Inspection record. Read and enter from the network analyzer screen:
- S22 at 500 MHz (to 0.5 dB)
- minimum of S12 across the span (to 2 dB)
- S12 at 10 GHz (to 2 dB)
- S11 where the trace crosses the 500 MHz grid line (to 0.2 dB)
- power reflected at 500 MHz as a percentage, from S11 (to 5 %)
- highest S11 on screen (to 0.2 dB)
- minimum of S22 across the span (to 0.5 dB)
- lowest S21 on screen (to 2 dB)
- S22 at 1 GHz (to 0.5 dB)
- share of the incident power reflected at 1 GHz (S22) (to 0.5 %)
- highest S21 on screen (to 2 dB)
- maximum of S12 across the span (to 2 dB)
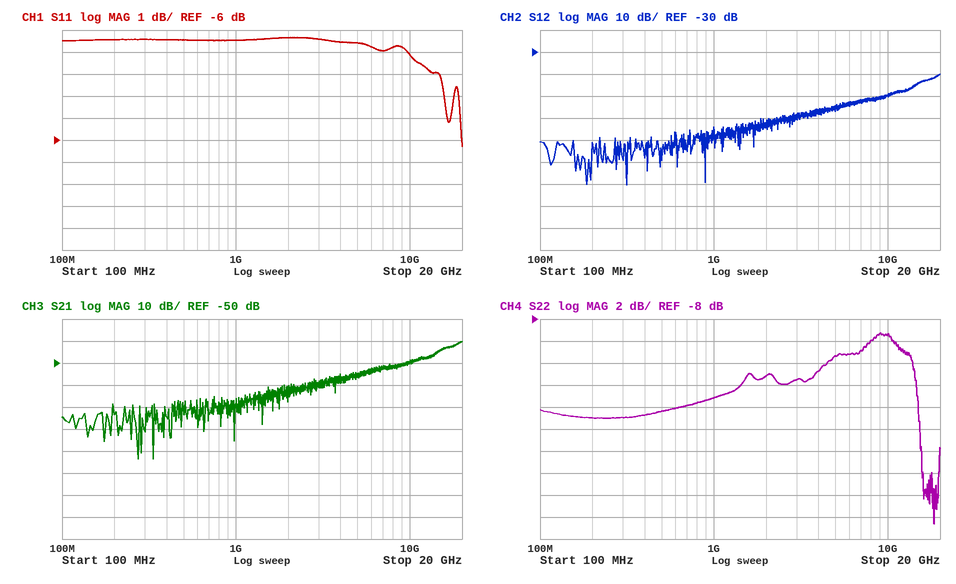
-16.5 dB
-90 dB
-50 dB
-1.4 dB
70 %
-1.4 dB
-26.5 dB
-94 dB
-15.0 dB
3.0 %
-40 dB
-40 dB
